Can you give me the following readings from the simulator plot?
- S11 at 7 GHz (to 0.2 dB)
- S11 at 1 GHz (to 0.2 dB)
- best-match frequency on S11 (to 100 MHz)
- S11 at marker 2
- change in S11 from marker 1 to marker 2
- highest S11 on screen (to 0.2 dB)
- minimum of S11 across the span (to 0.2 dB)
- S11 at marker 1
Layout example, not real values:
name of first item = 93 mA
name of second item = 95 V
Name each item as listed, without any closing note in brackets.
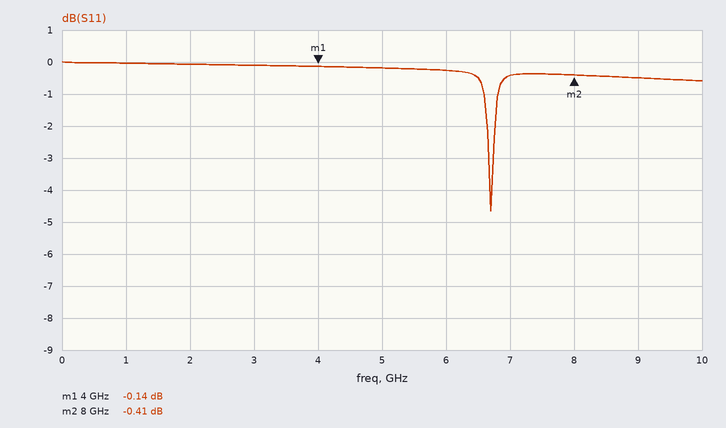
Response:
S11 at 7 GHz = -0.4 dB
S11 at 1 GHz = 0.0 dB
best-match frequency on S11 = 6.7 GHz
S11 at marker 2 = -0.41 dB
change in S11 from marker 1 to marker 2 = -0.27 dB
highest S11 on screen = 0.0 dB
minimum of S11 across the span = -4.6 dB
S11 at marker 1 = -0.14 dB
